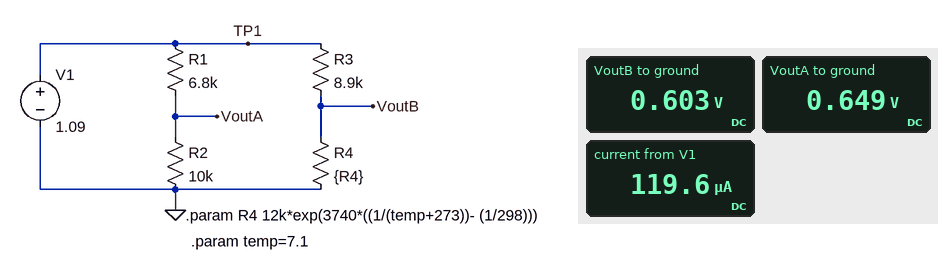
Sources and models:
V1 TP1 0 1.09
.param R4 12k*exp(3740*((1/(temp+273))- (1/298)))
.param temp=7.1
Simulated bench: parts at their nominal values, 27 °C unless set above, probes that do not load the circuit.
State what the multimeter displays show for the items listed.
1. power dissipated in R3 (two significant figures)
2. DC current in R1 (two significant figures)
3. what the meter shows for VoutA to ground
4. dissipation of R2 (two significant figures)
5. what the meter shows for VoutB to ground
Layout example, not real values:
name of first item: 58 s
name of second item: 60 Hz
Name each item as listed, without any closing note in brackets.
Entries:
power dissipated in R3: 27 µW
DC current in R1: 65 µA
what the meter shows for VoutA to ground: 0.649 V
dissipation of R2: 42 µW
what the meter shows for VoutB to ground: 0.603 V
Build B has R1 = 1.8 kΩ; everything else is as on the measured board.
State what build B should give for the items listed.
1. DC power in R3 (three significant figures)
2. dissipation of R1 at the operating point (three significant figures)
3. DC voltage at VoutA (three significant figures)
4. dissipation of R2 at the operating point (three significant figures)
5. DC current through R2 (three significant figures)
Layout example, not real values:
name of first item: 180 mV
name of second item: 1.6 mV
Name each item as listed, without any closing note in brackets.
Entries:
DC power in R3: 26.6 µW
dissipation of R1 at the operating point: 15.4 µW
DC voltage at VoutA: 924 mV
dissipation of R2 at the operating point: 85.3 µW
DC current through R2: 92.4 µA
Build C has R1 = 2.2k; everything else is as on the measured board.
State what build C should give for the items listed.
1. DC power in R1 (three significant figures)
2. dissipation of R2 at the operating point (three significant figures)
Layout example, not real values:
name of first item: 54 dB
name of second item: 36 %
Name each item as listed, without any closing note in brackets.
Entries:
DC power in R1: 17.6 µW
dissipation of R2 at the operating point: 79.8 µW
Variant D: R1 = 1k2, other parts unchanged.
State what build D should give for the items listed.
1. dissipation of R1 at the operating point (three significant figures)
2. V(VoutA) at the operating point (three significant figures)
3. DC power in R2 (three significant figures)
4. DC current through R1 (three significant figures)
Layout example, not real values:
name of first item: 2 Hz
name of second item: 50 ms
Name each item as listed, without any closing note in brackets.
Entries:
dissipation of R1 at the operating point: 11.4 µW
V(VoutA) at the operating point: 973 mV
DC power in R2: 94.7 µW
DC current through R1: 97.3 µA
